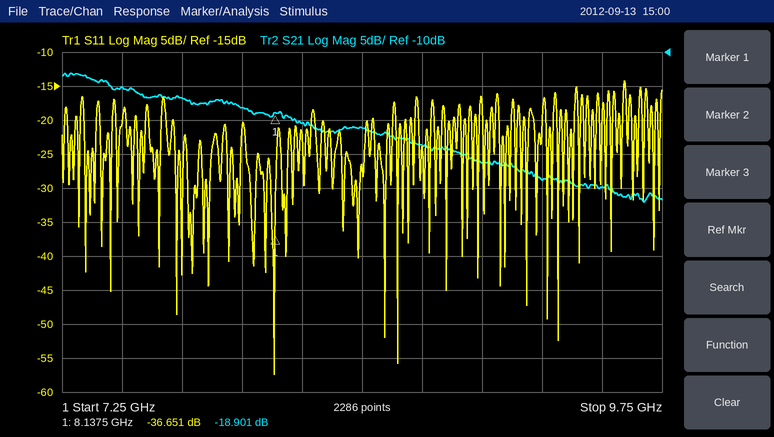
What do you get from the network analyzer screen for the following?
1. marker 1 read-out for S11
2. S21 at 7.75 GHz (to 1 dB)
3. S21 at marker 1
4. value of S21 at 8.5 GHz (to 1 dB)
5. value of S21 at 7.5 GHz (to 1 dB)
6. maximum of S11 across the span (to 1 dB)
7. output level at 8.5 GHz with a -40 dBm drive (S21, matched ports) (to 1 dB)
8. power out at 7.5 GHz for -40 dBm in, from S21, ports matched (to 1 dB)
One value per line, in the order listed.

-36.651 dB
-17 dB
-18.901 dB
-21 dB
-15 dB
-14 dB
-61 dBm
-55 dBm
